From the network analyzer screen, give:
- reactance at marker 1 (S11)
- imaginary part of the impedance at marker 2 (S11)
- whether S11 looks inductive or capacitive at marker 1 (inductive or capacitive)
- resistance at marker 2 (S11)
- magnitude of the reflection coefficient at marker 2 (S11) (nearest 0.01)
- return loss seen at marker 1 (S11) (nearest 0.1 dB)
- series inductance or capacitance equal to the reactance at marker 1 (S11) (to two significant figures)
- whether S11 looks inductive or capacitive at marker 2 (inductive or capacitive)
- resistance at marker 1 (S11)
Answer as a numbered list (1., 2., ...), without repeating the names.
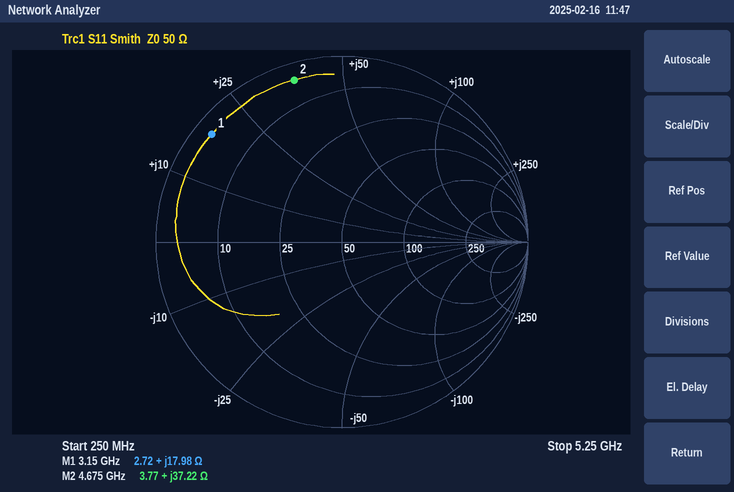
1. +17.98 Ω
2. +37.22 Ω
3. inductive
4. 3.77 Ω
5. 0.91
6. 0.8 dB
7. 910 pH
8. inductive
9. 2.72 Ω
